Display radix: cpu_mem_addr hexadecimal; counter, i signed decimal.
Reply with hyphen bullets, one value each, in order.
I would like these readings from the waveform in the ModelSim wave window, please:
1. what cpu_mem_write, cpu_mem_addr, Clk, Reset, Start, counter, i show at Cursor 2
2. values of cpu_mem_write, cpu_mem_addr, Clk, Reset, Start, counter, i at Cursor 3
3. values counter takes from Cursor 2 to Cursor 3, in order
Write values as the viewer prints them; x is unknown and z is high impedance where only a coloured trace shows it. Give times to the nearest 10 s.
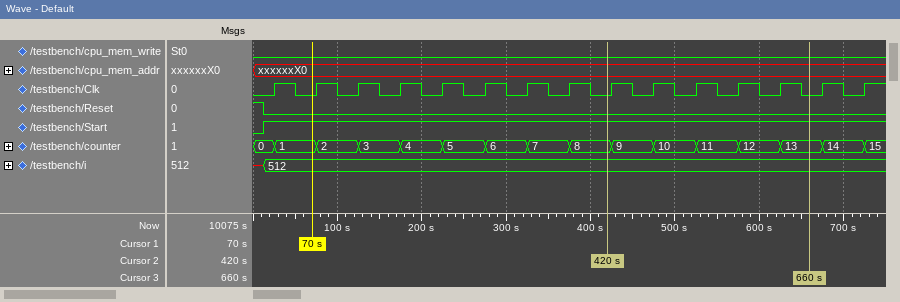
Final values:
- cpu_mem_write=0, cpu_mem_addr=xxxxxxX0, Clk=0, Reset=0, Start=1, counter=8, i=512
- cpu_mem_write=0, cpu_mem_addr=xxxxxxX0, Clk=0, Reset=0, Start=1, counter=13, i=512
- 8, 9, 10, 11, 12, 13
